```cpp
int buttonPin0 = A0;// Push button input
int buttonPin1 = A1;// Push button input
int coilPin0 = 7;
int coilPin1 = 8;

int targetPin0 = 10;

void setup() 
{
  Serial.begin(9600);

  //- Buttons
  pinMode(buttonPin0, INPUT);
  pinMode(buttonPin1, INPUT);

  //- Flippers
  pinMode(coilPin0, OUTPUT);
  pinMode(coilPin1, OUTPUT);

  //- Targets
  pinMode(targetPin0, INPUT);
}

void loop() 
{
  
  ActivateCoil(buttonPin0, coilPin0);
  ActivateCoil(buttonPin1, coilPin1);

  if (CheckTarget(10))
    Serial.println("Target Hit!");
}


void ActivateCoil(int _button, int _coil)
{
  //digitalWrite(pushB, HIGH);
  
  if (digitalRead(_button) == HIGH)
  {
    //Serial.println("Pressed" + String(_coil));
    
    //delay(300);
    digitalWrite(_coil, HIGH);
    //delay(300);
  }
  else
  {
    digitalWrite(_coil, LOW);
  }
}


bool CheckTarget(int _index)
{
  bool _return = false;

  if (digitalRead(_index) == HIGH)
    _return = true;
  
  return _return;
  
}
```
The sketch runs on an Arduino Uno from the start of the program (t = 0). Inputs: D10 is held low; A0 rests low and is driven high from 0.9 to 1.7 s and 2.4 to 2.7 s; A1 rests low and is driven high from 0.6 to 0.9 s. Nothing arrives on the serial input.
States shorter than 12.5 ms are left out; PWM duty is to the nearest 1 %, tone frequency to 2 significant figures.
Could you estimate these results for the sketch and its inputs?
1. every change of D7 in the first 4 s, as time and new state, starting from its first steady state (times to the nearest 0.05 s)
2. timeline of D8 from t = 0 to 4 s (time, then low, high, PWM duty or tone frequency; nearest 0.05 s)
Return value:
0 s low; 0.9 s high; 1.7 s low; 2.4 s high; 2.7 s low
0 s low; 0.6 s high; 0.9 s low
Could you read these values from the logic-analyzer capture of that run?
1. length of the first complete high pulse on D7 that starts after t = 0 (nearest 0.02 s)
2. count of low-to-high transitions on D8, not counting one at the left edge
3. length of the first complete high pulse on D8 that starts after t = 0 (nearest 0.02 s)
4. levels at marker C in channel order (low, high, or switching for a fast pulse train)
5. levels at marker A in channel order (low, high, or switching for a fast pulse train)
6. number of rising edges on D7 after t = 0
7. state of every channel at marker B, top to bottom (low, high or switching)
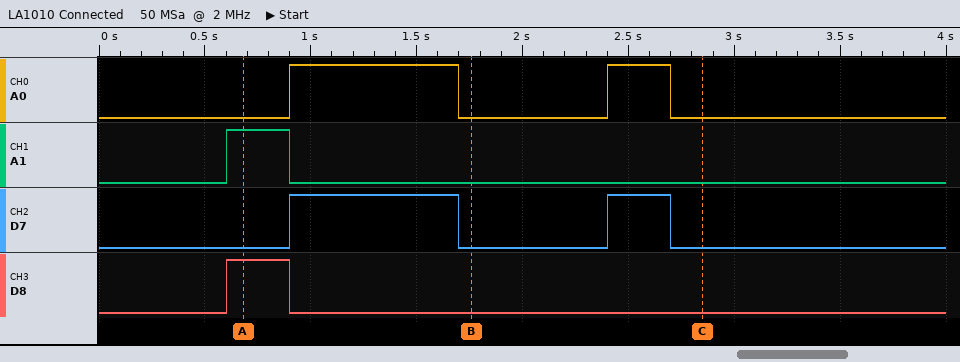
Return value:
0.80 s
1
0.30 s
A0 low, A1 low, D7 low, D8 low
A0 low, A1 high, D7 low, D8 high
2
A0 low, A1 low, D7 low, D8 low
